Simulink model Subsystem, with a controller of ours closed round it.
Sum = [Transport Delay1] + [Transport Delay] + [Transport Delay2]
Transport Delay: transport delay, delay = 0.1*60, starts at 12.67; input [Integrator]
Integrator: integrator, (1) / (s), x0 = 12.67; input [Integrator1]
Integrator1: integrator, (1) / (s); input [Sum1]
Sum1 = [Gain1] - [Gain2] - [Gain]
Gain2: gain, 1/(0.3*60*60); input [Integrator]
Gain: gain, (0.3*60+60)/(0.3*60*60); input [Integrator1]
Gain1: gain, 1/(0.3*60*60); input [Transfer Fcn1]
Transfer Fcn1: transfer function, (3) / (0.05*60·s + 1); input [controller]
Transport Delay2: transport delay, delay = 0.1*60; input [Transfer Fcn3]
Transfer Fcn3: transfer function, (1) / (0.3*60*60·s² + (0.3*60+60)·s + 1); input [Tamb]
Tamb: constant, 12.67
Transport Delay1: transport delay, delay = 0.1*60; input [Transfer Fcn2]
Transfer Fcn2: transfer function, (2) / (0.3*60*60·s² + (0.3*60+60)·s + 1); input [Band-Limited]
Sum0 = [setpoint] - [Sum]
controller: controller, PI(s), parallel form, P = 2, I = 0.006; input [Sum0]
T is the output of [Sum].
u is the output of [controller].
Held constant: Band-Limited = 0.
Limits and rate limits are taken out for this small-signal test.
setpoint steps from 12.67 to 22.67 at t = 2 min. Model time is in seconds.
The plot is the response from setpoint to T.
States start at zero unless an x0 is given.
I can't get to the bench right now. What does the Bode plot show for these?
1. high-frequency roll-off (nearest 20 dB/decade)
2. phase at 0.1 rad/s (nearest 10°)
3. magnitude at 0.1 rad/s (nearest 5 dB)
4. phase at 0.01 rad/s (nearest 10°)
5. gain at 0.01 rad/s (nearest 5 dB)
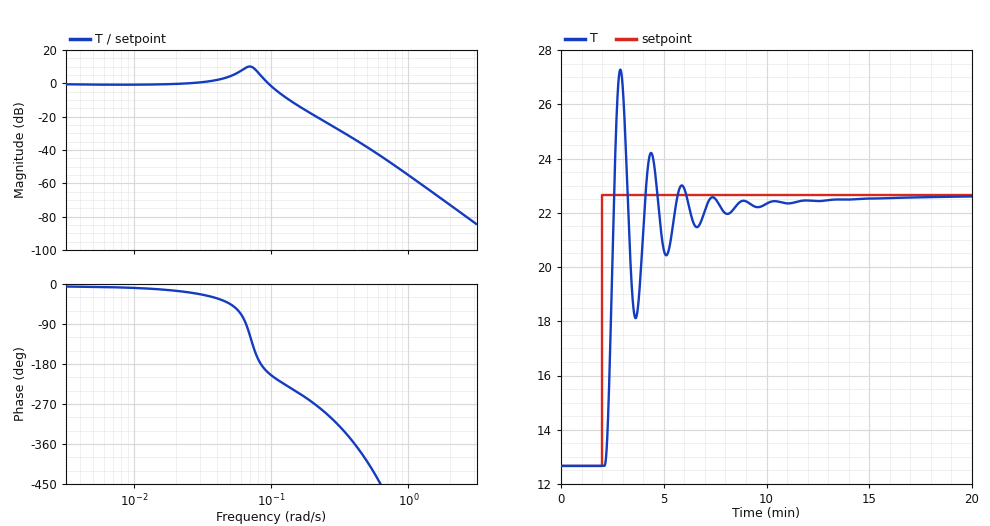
-60 dB/decade
-210°
0 dB
-10°
0 dB
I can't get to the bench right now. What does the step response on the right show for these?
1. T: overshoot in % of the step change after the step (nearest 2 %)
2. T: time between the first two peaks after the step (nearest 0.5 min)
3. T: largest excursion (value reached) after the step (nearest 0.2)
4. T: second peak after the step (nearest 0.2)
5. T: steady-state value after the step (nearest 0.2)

46 %
1.5 min
27.2
24.2
22.6
